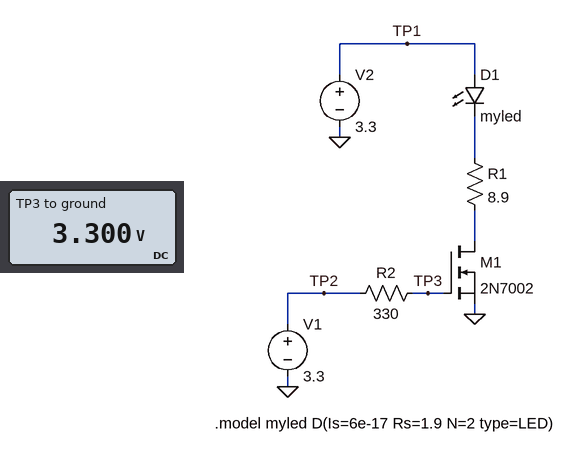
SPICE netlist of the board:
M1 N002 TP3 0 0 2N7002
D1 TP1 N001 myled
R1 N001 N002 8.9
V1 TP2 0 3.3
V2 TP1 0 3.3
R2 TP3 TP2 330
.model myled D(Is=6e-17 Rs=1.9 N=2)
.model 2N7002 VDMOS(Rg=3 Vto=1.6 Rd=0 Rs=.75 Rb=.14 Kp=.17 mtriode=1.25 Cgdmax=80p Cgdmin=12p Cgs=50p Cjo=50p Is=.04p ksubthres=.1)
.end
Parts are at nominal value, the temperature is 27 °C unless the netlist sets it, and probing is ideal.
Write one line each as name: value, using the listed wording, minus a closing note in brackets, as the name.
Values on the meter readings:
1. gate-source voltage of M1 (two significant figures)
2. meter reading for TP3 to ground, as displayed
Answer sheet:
gate-source voltage of M1: 3.3 V
meter reading for TP3 to ground, as displayed: 3.300 V
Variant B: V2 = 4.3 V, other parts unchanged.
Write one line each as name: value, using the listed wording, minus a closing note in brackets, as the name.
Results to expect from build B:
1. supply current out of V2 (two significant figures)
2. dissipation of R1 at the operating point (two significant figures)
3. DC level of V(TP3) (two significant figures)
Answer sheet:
supply current out of V2: 160 mA
dissipation of R1 at the operating point: 220 mW
DC level of V(TP3): 3.3 V
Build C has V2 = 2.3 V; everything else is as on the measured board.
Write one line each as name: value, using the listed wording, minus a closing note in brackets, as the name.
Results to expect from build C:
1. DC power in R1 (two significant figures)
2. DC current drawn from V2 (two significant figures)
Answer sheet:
DC power in R1: 12 mW
DC current drawn from V2: 37 mA
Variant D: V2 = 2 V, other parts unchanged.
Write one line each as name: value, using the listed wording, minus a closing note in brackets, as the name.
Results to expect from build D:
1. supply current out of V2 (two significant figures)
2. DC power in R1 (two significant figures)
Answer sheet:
supply current out of V2: 19 mA
DC power in R1: 3.2 mW
